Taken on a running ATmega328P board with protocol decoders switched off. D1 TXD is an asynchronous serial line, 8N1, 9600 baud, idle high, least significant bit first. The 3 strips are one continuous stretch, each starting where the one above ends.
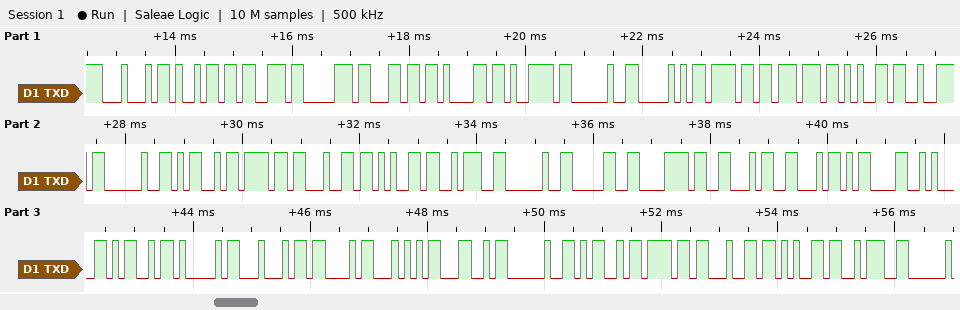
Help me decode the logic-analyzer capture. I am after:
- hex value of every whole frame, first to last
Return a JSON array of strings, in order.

["44 69 73 70 6C 61 79 20 50 6F 77 65 72 20 4D 6F 64 65 3A 20 30 78 46 46 0D 0A 4D 41 44 43 54 4C 20 4D 6F 64 65 3A"]
